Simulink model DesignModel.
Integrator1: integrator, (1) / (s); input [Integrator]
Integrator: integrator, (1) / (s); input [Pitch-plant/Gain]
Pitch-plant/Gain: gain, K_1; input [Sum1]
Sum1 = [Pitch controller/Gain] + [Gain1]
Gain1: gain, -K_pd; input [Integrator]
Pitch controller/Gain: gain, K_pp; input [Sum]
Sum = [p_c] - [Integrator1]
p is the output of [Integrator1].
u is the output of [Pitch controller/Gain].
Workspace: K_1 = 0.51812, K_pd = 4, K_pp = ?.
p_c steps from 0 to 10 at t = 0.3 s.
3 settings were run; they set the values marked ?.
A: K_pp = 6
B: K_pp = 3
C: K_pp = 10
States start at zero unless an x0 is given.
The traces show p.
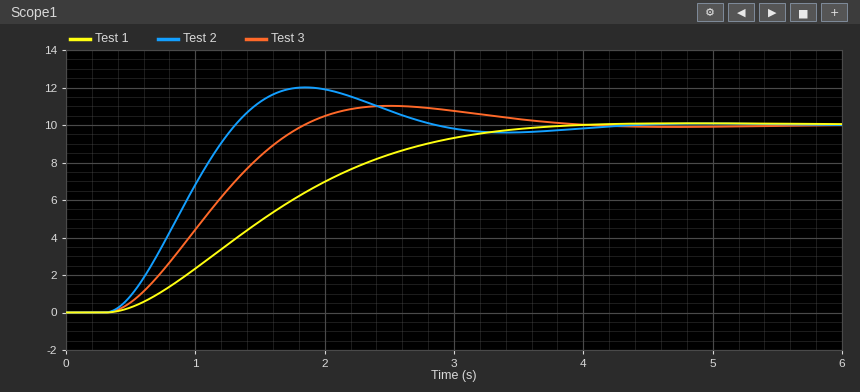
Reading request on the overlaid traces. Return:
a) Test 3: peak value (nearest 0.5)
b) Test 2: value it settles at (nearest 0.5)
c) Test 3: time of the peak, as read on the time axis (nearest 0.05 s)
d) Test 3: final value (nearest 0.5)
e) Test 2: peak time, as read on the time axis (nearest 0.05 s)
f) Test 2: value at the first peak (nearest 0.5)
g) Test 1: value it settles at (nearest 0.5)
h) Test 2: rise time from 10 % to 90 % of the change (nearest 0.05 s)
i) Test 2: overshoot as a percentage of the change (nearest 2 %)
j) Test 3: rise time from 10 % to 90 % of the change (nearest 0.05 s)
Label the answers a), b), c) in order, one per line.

a) 11.0
b) 10.0
c) 2.50 s
d) 10.0
e) 1.85 s
f) 12.0
g) 10.0
h) 0.70 s
i) 20 %
j) 1.05 s
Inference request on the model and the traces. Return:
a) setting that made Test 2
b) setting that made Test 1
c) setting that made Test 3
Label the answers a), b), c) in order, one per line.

a) C
b) B
c) A
